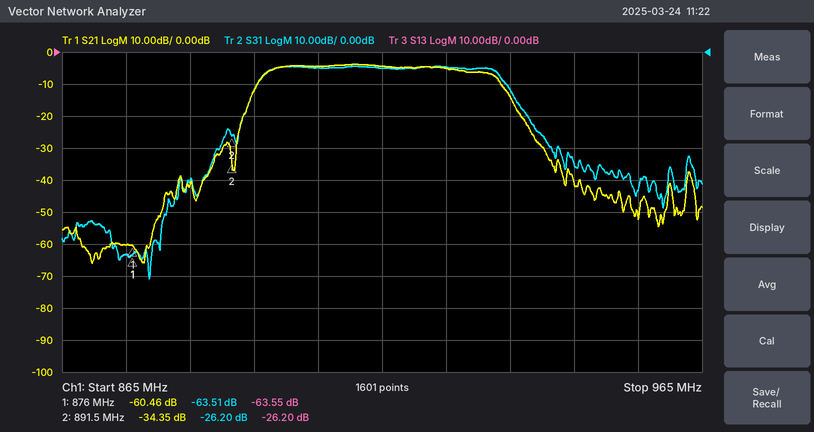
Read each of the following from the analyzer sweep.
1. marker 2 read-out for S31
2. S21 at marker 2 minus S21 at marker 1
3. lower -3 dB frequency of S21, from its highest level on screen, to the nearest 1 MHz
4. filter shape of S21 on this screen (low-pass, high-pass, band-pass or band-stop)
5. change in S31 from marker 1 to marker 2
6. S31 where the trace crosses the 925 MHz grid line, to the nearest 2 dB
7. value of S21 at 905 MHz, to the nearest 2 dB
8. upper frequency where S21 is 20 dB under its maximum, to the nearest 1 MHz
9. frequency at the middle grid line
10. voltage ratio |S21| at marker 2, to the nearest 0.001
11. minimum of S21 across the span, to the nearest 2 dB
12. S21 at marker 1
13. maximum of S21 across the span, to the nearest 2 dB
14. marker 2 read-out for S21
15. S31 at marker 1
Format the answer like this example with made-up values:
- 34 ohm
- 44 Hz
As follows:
- -26.20 dB
- 26.11 dB
- 897 MHz
- band-pass
- 37.31 dB
- -4 dB
- -4 dB
- 938 MHz
- 915 MHz
- 0.019
- -66 dB
- -60.46 dB
- -4 dB
- -34.35 dB
- -63.51 dB
